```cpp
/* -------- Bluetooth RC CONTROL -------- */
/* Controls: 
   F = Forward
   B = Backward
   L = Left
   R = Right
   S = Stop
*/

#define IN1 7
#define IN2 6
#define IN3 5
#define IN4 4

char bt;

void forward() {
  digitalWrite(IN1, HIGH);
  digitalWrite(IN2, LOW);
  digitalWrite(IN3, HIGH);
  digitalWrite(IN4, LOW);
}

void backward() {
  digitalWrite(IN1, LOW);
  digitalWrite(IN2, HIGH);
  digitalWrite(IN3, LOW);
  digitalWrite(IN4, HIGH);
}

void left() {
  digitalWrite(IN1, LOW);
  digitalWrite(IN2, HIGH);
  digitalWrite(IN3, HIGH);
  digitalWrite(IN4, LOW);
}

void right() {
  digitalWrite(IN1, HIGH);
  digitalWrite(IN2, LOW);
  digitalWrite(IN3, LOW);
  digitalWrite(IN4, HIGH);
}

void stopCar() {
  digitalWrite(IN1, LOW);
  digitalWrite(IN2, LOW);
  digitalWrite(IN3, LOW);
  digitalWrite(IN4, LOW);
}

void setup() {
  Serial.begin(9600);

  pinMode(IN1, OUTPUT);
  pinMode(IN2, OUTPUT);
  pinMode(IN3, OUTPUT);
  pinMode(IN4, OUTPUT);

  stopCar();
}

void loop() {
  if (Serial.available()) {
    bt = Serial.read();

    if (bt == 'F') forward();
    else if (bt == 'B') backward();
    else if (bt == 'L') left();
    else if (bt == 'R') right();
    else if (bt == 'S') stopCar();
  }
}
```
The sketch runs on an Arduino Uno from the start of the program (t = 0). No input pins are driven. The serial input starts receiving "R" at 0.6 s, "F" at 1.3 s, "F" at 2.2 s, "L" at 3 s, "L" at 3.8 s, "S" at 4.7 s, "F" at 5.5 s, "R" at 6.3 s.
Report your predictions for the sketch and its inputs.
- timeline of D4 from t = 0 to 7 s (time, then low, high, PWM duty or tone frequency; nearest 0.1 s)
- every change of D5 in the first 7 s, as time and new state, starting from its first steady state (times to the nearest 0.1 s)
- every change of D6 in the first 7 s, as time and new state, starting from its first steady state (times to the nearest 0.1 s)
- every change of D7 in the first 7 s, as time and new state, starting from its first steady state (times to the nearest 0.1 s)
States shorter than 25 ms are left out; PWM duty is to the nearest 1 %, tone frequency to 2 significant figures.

0 s low; 0.6 s high; 1.3 s low; 6.3 s high
0 s low; 1.3 s high; 4.7 s low; 5.5 s high; 6.3 s low
0 s low; 3 s high; 4.7 s low
0 s low; 0.6 s high; 3 s low; 5.5 s high
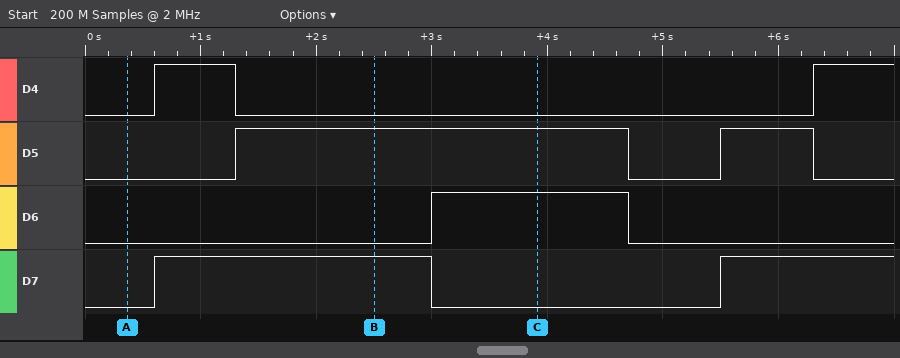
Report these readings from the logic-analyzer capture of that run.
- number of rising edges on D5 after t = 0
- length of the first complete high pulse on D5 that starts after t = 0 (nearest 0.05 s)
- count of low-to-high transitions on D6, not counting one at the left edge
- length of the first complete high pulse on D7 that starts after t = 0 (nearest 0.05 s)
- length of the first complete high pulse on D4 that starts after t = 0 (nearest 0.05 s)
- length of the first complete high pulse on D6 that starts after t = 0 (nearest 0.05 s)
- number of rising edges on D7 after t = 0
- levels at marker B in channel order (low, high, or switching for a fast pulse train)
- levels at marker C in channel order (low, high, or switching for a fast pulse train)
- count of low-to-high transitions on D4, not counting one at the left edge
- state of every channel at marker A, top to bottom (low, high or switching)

2
3.40 s
1
2.40 s
0.70 s
1.70 s
2
D4 low, D5 high, D6 low, D7 high
D4 low, D5 high, D6 high, D7 low
2
D4 low, D5 low, D6 low, D7 low
